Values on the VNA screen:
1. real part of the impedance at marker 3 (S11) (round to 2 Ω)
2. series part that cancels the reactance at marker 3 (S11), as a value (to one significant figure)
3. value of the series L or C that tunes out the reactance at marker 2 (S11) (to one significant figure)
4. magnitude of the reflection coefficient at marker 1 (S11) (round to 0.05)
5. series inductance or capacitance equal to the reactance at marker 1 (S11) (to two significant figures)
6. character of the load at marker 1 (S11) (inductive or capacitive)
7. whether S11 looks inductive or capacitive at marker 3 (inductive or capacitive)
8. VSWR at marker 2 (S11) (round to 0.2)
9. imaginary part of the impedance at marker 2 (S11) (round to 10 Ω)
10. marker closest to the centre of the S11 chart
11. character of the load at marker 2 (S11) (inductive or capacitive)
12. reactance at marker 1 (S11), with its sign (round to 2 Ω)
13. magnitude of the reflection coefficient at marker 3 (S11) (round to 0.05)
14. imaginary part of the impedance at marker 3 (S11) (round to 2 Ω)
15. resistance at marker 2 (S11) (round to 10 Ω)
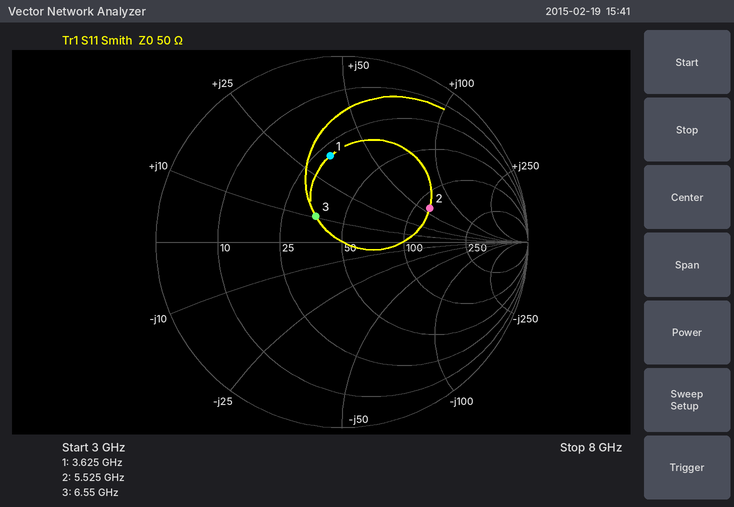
36 Ω
2 pF
500 fF
0.45
1.5 nH
inductive
inductive
3.0
+60 Ω
marker 3
inductive
+34 Ω
0.20
+10 Ω
120 Ω
